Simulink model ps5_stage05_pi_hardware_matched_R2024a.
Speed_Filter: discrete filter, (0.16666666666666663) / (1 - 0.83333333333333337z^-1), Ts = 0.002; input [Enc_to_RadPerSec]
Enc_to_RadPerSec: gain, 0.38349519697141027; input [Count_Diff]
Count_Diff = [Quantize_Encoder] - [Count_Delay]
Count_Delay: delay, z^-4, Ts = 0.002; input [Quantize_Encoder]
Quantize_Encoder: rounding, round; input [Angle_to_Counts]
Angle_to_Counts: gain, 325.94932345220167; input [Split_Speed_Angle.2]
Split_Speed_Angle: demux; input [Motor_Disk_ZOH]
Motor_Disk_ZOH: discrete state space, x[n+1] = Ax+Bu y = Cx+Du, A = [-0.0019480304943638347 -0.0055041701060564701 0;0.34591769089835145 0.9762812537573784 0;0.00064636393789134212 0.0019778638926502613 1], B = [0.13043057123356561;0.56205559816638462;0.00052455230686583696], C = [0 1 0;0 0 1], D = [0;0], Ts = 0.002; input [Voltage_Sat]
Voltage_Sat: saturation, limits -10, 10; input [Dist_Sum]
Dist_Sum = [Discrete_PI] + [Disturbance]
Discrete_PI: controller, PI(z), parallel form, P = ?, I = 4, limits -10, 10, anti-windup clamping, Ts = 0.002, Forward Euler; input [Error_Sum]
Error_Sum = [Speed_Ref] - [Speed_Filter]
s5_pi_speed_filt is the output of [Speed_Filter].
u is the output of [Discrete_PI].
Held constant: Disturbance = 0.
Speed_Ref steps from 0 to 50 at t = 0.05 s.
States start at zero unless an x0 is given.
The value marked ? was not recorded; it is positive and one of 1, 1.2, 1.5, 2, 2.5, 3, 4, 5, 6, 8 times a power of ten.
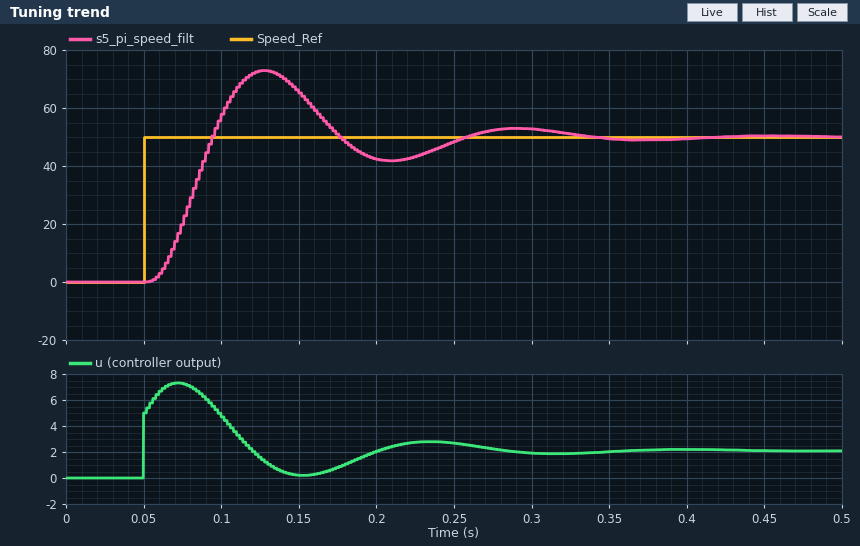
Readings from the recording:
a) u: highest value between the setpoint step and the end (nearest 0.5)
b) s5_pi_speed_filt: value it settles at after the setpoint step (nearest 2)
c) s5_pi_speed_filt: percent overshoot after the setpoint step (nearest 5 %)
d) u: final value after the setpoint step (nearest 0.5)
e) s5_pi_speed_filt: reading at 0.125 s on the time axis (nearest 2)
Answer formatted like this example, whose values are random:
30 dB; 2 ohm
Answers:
7.5; 50; 45 %; 2.0; 72
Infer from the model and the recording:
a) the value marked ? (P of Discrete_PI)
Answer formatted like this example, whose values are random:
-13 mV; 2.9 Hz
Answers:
0.1
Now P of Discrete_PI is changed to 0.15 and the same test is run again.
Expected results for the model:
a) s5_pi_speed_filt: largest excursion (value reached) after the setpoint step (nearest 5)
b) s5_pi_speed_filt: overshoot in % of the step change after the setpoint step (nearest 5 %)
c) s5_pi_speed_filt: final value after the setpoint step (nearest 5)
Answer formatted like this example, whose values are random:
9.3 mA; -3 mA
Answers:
70; 35 %; 50
